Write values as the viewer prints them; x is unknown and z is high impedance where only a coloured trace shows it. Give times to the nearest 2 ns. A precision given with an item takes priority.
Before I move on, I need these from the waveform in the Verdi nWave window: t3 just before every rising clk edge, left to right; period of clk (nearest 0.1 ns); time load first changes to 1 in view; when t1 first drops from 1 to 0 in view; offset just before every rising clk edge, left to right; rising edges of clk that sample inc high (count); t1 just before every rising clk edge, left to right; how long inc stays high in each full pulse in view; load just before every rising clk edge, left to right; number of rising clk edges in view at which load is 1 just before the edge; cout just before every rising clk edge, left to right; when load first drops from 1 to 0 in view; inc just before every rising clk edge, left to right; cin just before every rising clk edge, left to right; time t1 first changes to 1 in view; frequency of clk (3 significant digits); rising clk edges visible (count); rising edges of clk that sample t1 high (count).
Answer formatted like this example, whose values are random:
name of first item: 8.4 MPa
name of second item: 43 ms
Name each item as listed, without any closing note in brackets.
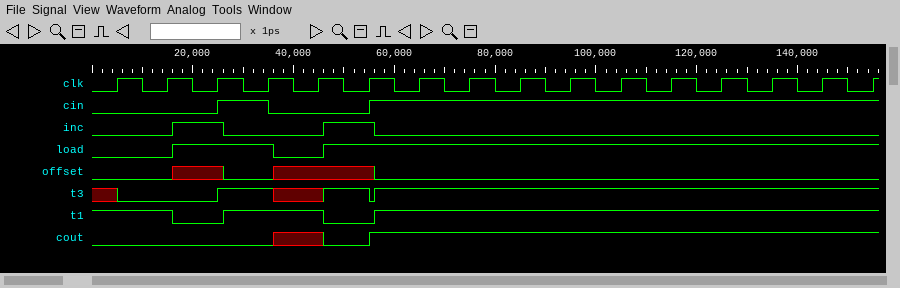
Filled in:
t3 just before every rising clk edge, left to right: x 0 0 1 x 1 1 1 1 1 1 1 1 1 1 1
period of clk: 10 ns
time load first changes to 1 in view: 16 ns
when t1 first drops from 1 to 0 in view: 16 ns
offset just before every rising clk edge, left to right: 0 0 x 0 x x 0 0 0 0 0 0 0 0 0 0
rising edges of clk that sample inc high: 2
t1 just before every rising clk edge, left to right: 1 1 0 1 1 0 1 1 1 1 1 1 1 1 1 1
how long inc stays high in each full pulse in view: 10 ns, 10 ns
load just before every rising clk edge, left to right: 0 0 1 1 0 1 1 1 1 1 1 1 1 1 1 1
number of rising clk edges in view at which load is 1 just before the edge: 13
cout just before every rising clk edge, left to right: 0 0 0 0 x 0 1 1 1 1 1 1 1 1 1 1
when load first drops from 1 to 0 in view: 36 ns
inc just before every rising clk edge, left to right: 0 0 1 0 0 1 0 0 0 0 0 0 0 0 0 0
cin just before every rising clk edge, left to right: 0 0 0 1 0 0 1 1 1 1 1 1 1 1 1 1
time t1 first changes to 1 in view: 26 ns
frequency of clk: 100 MHz
rising clk edges visible: 16
rising edges of clk that sample t1 high: 14
